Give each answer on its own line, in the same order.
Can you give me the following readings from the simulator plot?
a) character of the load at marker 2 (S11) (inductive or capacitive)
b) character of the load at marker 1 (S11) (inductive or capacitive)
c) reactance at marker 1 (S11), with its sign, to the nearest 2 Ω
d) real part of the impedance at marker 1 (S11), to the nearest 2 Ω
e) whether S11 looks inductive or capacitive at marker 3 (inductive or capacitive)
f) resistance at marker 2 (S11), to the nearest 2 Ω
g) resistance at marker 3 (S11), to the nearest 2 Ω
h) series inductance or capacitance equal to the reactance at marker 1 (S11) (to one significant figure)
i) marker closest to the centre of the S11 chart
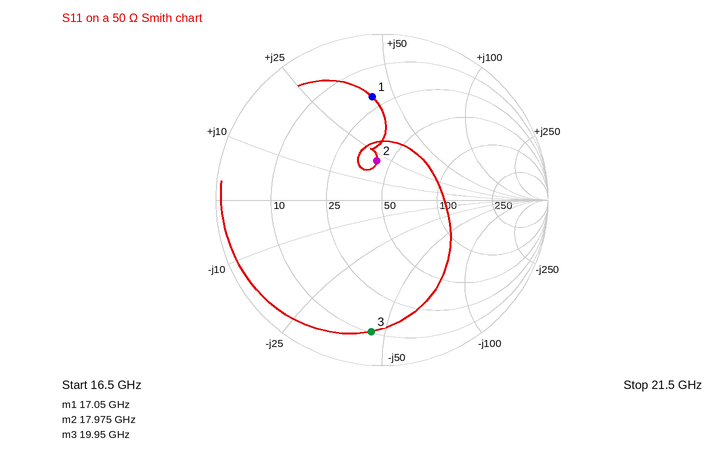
inductive
inductive
+42 Ω
20 Ω
capacitive
42 Ω
10 Ω
400 pH
marker 2
